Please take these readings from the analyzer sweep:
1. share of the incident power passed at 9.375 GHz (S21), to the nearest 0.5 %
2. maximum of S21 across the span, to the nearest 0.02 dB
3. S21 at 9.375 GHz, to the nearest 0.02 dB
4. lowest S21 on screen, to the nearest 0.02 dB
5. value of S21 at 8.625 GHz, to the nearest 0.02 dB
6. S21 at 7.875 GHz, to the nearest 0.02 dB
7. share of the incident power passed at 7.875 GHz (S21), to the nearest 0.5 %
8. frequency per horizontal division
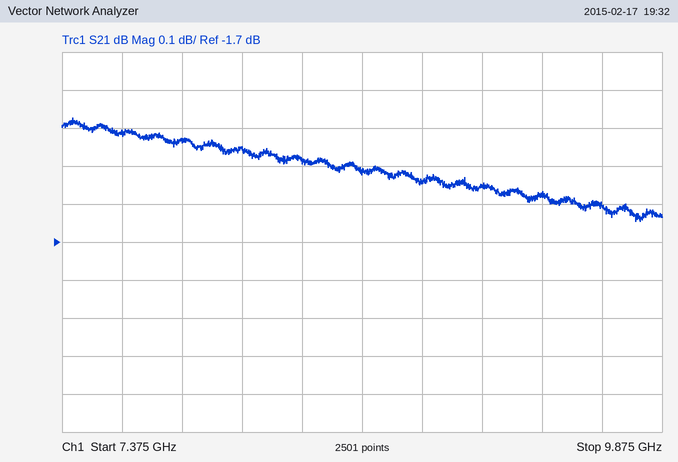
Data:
69.5 %
-1.38 dB
-1.58 dB
-1.64 dB
-1.52 dB
-1.44 dB
72.0 %
250 MHz
